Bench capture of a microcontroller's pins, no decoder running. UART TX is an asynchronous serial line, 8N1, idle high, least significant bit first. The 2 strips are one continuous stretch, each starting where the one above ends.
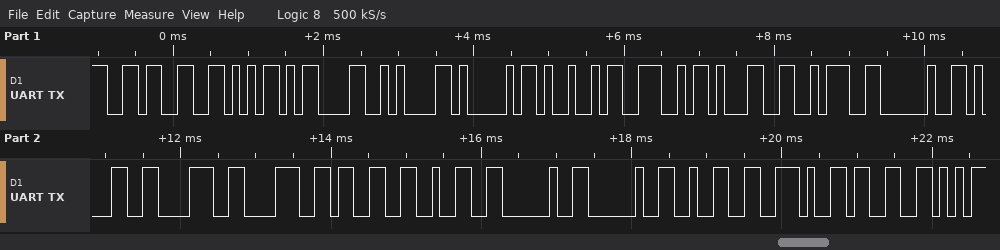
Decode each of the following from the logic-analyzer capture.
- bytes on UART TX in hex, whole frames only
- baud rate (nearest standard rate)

0x36 0x56 0x0D 0x0A 0x41 0x49 0x4E 0x31 0x3A 0x20 0x31 0x38 0x38 0x33 0x32 0x20 0x20 0x32 0x2E 0x33
9600 baud
